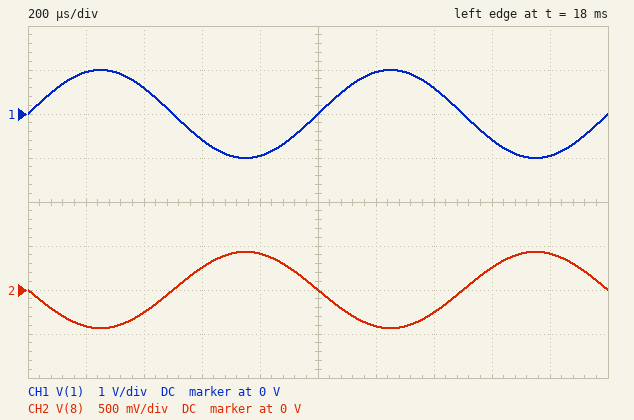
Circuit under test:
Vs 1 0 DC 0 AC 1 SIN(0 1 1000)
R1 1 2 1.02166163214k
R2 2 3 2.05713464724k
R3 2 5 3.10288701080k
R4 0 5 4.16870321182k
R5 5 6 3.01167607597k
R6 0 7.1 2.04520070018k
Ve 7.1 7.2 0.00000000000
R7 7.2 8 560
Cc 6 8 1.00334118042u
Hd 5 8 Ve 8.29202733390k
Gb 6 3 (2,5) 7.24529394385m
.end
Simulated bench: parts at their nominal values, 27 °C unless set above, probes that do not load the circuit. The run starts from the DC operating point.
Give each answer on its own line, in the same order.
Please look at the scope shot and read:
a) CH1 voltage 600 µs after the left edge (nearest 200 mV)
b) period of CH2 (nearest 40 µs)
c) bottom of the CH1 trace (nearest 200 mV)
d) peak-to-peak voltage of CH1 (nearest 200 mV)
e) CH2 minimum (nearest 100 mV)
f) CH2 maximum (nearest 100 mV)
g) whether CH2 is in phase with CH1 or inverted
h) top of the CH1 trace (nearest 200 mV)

-600 mV
1.00 ms
-1.0 V
2.0 V
-400 mV
400 mV
inverted
1.0 V
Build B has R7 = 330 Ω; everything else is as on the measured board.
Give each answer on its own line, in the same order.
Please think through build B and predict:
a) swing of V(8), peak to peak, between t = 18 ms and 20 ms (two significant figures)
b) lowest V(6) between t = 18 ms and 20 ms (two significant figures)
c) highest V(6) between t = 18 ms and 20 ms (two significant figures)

760 mV
-380 mV
380 mV
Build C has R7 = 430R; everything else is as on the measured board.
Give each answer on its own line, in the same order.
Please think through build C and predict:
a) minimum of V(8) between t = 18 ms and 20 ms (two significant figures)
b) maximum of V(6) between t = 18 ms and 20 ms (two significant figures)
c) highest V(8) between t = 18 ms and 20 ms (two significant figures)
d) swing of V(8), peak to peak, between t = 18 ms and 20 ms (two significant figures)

-400 mV
410 mV
400 mV
800 mV
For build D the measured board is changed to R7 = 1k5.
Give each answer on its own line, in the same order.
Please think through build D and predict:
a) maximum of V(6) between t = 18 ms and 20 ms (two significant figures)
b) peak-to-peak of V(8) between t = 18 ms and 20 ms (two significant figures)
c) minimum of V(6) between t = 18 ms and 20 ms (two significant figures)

730 mV
1.5 V
-730 mV
